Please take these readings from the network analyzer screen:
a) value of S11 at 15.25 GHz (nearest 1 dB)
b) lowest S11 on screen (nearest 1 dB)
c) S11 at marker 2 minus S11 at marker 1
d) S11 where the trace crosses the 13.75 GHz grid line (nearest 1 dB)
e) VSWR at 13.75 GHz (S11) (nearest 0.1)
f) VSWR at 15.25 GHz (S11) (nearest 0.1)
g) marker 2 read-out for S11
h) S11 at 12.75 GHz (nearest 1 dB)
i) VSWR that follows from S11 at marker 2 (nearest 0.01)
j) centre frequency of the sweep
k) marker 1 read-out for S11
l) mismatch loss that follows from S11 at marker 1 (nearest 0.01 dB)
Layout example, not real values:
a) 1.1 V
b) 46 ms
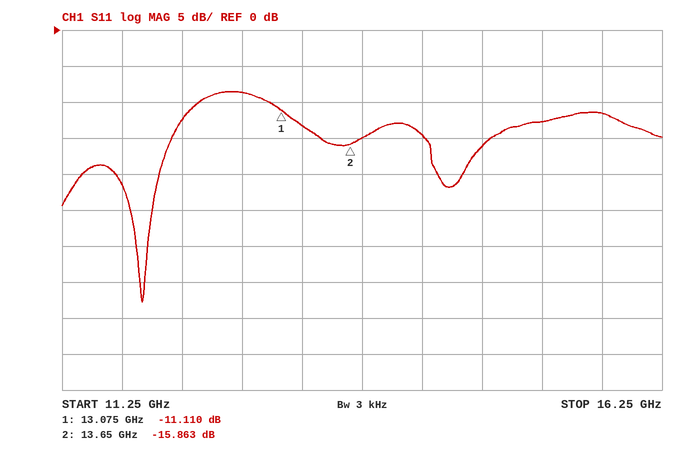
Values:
a) -13 dB
b) -38 dB
c) -4.753 dB
d) -15 dB
e) 1.4
f) 1.6
g) -15.863 dB
h) -9 dB
i) 1.38
j) 13.75 GHz
k) -11.110 dB
l) 0.35 dB
